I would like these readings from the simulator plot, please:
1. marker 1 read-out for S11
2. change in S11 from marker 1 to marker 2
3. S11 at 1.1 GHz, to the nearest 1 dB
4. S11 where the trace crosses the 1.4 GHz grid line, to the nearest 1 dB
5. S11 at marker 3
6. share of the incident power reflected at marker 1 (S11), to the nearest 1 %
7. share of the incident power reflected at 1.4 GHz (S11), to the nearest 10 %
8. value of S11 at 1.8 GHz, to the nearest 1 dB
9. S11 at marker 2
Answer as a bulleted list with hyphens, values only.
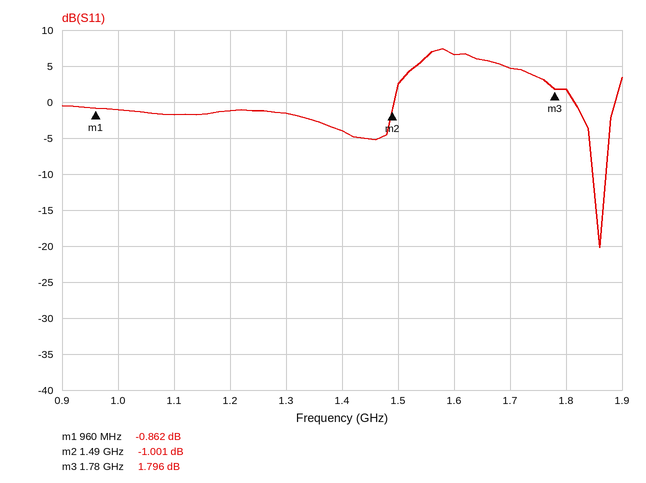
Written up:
- -0.862 dB
- -0.139 dB
- -2 dB
- -4 dB
- 1.796 dB
- 82 %
- 40 %
- 2 dB
- -1.001 dB
